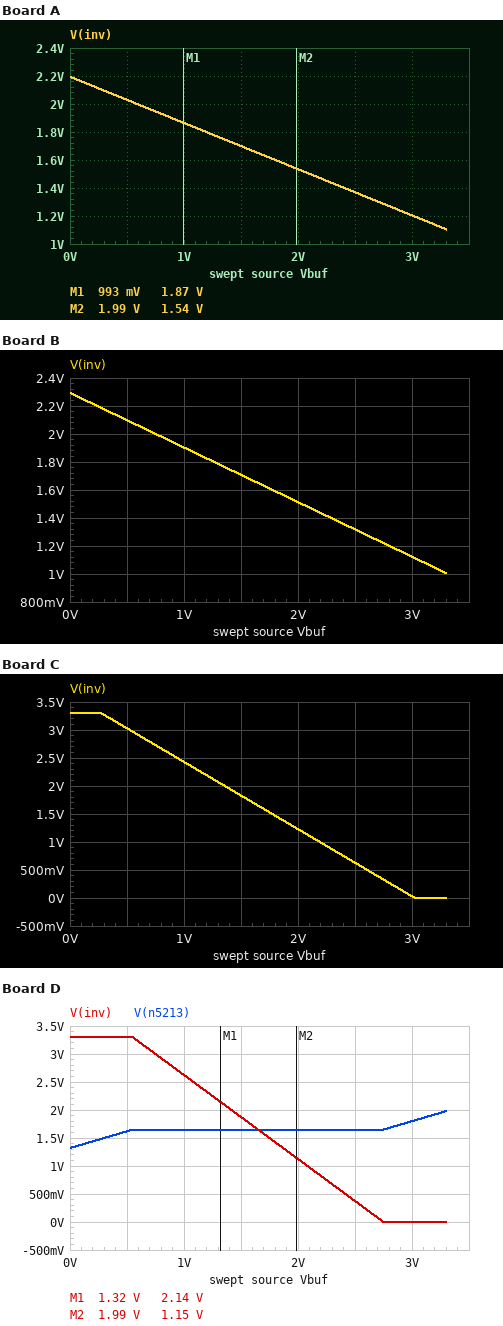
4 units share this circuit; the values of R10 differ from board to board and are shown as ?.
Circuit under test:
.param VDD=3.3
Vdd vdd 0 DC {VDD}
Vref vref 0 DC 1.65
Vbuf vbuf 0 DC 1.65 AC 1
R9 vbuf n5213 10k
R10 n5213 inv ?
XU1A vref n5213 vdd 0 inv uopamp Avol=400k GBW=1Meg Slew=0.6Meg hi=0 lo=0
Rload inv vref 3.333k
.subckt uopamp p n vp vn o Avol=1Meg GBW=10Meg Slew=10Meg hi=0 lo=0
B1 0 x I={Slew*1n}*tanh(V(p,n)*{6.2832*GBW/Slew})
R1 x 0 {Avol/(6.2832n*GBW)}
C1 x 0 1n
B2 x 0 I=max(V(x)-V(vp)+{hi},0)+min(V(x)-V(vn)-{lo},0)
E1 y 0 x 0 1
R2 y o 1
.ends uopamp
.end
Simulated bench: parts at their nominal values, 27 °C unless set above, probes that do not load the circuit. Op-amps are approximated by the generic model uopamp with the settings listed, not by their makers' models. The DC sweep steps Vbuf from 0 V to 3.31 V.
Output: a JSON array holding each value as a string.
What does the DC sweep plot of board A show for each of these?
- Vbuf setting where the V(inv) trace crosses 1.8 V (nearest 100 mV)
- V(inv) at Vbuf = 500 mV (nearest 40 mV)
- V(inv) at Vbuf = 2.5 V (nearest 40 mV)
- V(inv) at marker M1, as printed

["1.2 V", "2.04 V", "1.36 V", "1.87 V"]
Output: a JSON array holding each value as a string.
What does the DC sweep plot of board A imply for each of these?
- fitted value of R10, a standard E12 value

["3.3 kΩ"]
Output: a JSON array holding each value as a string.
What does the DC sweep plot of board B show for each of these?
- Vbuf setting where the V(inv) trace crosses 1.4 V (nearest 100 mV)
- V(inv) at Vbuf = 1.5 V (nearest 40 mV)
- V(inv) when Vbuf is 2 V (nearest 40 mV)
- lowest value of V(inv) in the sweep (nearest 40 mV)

["2.3 V", "1.72 V", "1.52 V", "1.00 V"]
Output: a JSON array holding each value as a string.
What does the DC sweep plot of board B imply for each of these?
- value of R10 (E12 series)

["3.9 kΩ"]
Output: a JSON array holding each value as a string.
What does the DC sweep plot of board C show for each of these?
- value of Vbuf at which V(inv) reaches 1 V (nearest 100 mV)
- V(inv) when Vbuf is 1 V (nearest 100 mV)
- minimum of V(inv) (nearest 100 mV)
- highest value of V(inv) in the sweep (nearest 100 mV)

["2.2 V", "2.4 V", "0 V", "3.3 V"]
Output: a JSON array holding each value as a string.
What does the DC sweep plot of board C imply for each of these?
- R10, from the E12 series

["12 kΩ"]
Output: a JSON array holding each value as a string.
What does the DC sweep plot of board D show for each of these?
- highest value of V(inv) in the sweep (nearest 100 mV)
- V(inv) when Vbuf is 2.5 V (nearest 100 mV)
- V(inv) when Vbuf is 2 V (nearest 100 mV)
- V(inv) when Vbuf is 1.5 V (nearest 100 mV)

["3.3 V", "400 mV", "1.1 V", "1.9 V"]
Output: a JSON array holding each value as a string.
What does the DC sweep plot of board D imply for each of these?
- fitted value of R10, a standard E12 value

["15 kΩ"]
